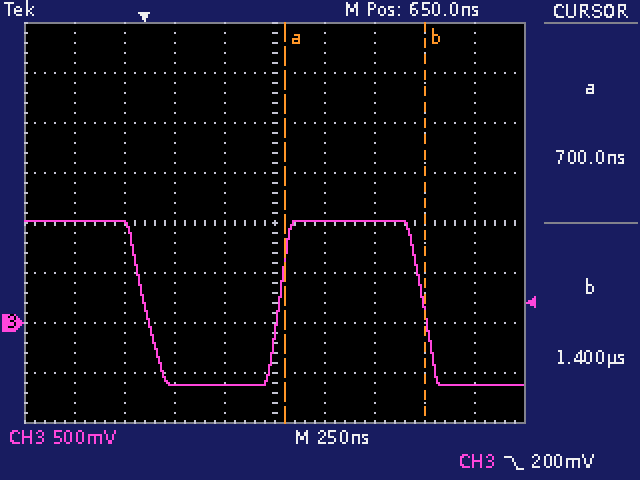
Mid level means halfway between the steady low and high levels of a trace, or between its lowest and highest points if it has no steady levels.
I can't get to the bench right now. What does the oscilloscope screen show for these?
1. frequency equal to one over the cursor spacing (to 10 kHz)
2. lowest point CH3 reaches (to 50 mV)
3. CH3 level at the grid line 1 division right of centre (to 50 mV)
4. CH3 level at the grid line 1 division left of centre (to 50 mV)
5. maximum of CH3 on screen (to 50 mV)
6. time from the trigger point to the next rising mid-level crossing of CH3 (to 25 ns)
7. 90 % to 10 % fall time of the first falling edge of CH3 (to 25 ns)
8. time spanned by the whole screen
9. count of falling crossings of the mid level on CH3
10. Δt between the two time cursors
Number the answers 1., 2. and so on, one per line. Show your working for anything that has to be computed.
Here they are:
1. 1 / 700 ns ≈ 1.43 MHz
2. -600 mV
3. 1.00 V
4. -600 mV
5. 1.00 V
6. 675 ns
7. 150 ns
8. 2.5 µs
9. 2
10. 1.4 µs − (700 ns) = 700 ns
